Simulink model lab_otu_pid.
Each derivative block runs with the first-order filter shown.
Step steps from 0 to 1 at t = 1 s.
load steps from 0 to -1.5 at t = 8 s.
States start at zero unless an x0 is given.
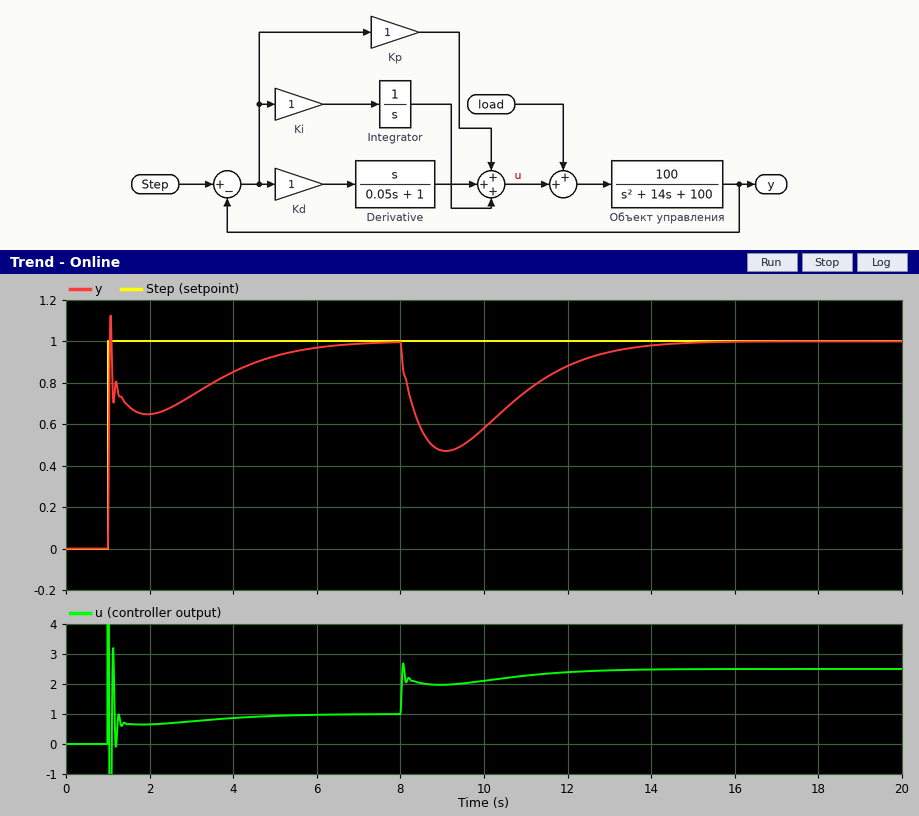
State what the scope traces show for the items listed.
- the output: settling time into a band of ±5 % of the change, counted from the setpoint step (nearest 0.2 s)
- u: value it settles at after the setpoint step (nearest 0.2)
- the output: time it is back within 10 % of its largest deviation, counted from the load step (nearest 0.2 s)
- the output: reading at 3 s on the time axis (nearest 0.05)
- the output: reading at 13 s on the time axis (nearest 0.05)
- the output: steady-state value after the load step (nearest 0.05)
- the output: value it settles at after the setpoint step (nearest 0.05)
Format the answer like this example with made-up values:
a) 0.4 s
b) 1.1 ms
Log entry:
a) 4.4 s
b) 1.0
c) 5.0 s
d) 0.75
e) 0.95
f) 1.00
g) 1.00
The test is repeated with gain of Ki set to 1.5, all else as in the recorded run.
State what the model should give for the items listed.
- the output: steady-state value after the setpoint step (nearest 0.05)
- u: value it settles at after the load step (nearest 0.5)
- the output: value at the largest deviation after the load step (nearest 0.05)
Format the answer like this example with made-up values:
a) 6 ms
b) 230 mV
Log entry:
a) 1.00
b) 2.5
c) 0.50
